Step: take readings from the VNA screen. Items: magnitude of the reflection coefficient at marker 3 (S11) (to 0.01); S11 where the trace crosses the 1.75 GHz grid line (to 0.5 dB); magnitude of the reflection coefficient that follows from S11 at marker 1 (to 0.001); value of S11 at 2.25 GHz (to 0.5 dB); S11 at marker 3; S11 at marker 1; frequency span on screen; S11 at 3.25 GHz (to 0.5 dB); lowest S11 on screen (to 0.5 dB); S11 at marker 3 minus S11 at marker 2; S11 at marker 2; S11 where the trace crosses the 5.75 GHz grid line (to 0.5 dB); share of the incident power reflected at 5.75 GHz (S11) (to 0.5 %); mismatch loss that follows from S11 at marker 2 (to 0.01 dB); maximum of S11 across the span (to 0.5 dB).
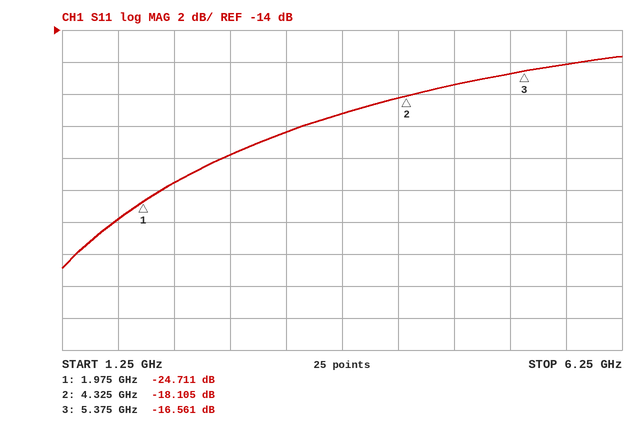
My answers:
0.15
-26.0 dB
0.058
-23.5 dB
-16.561 dB
-24.711 dB
5 GHz
-20.5 dB
-29.0 dB
1.544 dB
-18.105 dB
-16.0 dB
2.5 %
0.07 dB
-15.5 dB
